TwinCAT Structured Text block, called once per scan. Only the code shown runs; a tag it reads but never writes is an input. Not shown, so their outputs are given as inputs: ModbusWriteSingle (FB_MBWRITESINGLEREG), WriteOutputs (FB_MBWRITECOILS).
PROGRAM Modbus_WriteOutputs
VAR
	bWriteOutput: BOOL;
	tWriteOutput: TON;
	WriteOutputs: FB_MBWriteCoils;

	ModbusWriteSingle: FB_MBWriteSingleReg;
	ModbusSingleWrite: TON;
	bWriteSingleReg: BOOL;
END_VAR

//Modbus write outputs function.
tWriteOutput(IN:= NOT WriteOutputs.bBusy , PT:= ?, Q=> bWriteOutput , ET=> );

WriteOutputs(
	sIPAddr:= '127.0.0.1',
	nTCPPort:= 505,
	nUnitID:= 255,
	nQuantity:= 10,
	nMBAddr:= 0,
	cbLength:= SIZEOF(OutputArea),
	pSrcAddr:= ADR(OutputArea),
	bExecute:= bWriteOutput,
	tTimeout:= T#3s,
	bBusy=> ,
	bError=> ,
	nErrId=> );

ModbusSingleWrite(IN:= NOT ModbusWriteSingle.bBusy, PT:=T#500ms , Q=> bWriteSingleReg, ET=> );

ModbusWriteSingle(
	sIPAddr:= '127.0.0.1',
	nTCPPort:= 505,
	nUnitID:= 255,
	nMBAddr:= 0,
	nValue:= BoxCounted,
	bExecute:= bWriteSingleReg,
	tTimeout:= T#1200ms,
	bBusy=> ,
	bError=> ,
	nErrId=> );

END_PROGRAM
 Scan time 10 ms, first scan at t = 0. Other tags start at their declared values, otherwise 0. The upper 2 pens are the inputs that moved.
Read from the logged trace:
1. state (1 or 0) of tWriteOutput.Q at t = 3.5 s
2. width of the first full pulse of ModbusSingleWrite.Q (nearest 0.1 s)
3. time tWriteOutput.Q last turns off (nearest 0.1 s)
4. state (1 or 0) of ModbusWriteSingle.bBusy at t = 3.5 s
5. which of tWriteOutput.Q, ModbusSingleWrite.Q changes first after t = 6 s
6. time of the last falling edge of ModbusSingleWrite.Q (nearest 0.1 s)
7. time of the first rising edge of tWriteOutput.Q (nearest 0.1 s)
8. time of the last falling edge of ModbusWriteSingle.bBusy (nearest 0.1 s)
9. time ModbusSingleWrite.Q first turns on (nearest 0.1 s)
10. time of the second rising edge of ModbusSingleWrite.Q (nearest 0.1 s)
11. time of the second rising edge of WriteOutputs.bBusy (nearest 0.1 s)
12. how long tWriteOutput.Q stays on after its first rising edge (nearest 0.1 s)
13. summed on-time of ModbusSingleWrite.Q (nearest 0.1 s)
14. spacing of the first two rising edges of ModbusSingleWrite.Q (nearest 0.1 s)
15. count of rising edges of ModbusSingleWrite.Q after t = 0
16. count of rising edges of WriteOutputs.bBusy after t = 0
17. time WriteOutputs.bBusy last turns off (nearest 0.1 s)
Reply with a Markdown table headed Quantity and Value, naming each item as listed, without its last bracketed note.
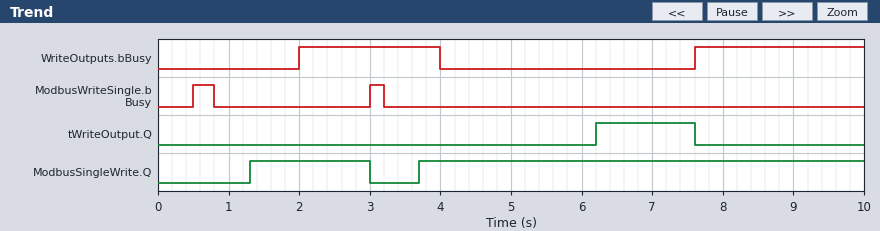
| Quantity | Value |
|---|---|
| state (1 or 0) of tWriteOutput.Q at t = 3.5 s | 0 |
| width of the first full pulse of ModbusSingleWrite.Q | 1.7 s |
| time tWriteOutput.Q last turns off | 7.6 s |
| state (1 or 0) of ModbusWriteSingle.bBusy at t = 3.5 s | 0 |
| which of tWriteOutput.Q, ModbusSingleWrite.Q changes first after t = 6 s | tWriteOutput.Q |
| time of the last falling edge of ModbusSingleWrite.Q | 3.0 s |
| time of the first rising edge of tWriteOutput.Q | 6.2 s |
| time of the last falling edge of ModbusWriteSingle.bBusy | 3.2 s |
| time ModbusSingleWrite.Q first turns on | 1.3 s |
| time of the second rising edge of ModbusSingleWrite.Q | 3.7 s |
| time of the second rising edge of WriteOutputs.bBusy | 7.6 s |
| how long tWriteOutput.Q stays on after its first rising edge | 1.4 s |
| summed on-time of ModbusSingleWrite.Q | 8.0 s |
| spacing of the first two rising edges of ModbusSingleWrite.Q | 2.4 s |
| count of rising edges of ModbusSingleWrite.Q after t = 0 | 2 |
| count of rising edges of WriteOutputs.bBusy after t = 0 | 2 |
| time WriteOutputs.bBusy last turns off | 4.0 s |
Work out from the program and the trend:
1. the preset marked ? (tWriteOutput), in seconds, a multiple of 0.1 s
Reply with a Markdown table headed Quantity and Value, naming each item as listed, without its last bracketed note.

| Quantity | Value |
|---|---|
| the preset marked ? (tWriteOutput), in seconds, a multiple of 0.1 s | 2.2 s |
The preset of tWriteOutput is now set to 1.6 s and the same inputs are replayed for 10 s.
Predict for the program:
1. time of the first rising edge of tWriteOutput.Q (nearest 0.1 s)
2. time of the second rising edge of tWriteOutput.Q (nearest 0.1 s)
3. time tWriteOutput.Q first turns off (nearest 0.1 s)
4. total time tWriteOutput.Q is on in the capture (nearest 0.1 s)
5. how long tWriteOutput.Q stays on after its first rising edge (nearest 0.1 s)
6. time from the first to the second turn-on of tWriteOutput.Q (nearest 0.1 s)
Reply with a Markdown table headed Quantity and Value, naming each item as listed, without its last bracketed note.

| Quantity | Value |
|---|---|
| time of the first rising edge of tWriteOutput.Q | 1.6 s |
| time of the second rising edge of tWriteOutput.Q | 5.6 s |
| time tWriteOutput.Q first turns off | 2.0 s |
| total time tWriteOutput.Q is on in the capture | 2.4 s |
| how long tWriteOutput.Q stays on after its first rising edge | 0.4 s |
| time from the first to the second turn-on of tWriteOutput.Q | 4.0 s |
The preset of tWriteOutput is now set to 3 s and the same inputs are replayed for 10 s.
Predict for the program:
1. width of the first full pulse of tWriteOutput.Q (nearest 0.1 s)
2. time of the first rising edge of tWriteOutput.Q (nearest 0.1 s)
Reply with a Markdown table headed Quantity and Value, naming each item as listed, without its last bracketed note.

| Quantity | Value |
|---|---|
| width of the first full pulse of tWriteOutput.Q | 0.6 s |
| time of the first rising edge of tWriteOutput.Q | 7.0 s |
